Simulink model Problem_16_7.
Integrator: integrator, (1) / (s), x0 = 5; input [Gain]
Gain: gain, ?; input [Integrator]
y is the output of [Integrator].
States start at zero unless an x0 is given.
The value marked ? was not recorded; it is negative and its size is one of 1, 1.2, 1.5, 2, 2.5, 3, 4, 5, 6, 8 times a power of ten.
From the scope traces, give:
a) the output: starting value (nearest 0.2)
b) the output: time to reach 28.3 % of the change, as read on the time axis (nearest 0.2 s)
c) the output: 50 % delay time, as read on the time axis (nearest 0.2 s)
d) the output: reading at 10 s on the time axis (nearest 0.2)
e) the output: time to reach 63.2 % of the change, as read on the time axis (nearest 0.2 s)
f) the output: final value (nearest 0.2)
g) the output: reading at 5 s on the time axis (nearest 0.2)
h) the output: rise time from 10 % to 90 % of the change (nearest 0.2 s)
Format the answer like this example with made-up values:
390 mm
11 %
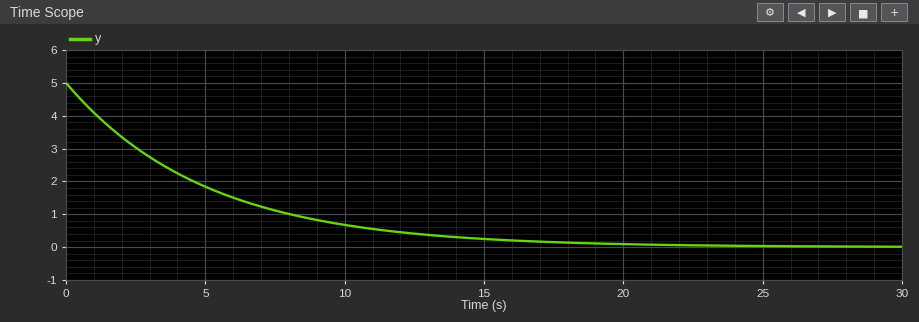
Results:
5.0
1.6 s
3.4 s
0.6
5.0 s
0.0
1.8
11.0 s
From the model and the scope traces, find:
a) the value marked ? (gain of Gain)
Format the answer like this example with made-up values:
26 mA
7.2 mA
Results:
-0.2
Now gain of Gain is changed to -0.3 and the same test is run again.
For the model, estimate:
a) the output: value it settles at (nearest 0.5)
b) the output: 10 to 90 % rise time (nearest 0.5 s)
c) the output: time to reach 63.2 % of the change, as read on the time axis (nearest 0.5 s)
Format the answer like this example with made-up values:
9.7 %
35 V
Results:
0.0
7.5 s
3.5 s
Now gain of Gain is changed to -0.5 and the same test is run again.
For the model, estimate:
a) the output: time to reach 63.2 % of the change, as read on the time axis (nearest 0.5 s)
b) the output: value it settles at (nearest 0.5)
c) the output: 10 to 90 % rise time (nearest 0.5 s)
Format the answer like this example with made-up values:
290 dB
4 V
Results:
2.0 s
0.0
4.5 s
